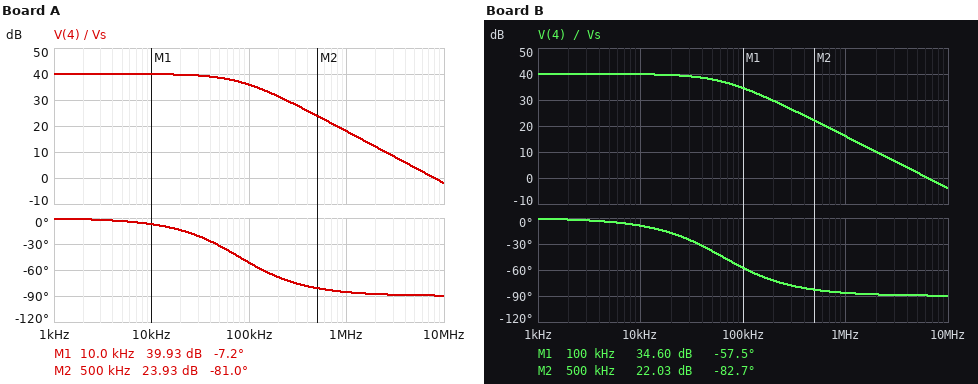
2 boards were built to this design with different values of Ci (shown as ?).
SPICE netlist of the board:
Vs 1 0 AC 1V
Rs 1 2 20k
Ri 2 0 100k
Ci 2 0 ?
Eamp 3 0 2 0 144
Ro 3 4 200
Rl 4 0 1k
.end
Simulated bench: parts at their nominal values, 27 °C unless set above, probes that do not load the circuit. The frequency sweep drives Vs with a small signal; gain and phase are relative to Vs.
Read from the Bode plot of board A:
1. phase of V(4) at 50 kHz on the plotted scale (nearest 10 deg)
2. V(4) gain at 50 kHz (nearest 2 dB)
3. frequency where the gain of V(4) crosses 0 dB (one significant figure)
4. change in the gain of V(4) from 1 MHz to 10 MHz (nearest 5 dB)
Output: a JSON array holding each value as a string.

["-30 deg", "38 dB", "8 MHz", "-20 dB"]
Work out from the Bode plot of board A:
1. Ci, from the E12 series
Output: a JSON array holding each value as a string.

["120 pF"]
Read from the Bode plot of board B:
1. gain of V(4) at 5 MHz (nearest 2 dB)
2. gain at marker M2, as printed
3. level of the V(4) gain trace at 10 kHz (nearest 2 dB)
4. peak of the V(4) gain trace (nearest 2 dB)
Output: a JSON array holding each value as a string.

["2 dB", "22.03 dB", "40 dB", "40 dB"]
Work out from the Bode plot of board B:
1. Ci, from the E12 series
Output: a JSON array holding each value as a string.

["150 pF"]
